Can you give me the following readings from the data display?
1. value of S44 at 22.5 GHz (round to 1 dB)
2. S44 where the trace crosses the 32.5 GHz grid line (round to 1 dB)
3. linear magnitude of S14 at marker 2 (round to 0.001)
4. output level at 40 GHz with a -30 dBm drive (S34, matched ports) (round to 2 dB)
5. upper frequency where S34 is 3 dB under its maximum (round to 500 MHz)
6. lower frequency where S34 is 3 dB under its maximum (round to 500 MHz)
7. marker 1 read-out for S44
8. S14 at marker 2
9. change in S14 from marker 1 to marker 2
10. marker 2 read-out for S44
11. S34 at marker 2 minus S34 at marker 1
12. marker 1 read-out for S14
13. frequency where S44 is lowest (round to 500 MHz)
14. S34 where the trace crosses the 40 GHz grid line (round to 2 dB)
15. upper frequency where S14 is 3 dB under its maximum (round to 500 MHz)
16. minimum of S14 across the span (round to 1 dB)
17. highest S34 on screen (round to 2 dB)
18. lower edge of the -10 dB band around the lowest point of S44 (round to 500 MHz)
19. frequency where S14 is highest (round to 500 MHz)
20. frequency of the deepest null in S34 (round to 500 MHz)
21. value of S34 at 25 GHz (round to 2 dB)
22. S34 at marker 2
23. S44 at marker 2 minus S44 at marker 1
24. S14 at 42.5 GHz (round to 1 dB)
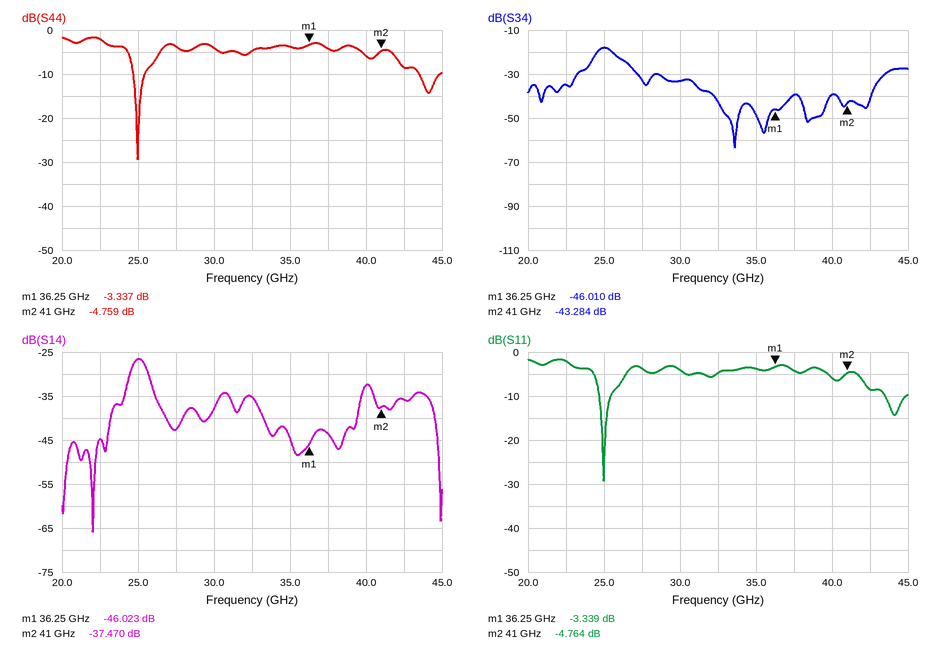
-2 dB
-5 dB
0.013
-70 dBm
25.5 GHz
24.5 GHz
-3.337 dB
-37.470 dB
8.553 dB
-4.759 dB
2.726 dB
-46.023 dB
25.0 GHz
-40 dB
25.5 GHz
-66 dB
-18 dB
24.5 GHz
25.0 GHz
33.5 GHz
-18 dB
-43.284 dB
-1.422 dB
-36 dB
